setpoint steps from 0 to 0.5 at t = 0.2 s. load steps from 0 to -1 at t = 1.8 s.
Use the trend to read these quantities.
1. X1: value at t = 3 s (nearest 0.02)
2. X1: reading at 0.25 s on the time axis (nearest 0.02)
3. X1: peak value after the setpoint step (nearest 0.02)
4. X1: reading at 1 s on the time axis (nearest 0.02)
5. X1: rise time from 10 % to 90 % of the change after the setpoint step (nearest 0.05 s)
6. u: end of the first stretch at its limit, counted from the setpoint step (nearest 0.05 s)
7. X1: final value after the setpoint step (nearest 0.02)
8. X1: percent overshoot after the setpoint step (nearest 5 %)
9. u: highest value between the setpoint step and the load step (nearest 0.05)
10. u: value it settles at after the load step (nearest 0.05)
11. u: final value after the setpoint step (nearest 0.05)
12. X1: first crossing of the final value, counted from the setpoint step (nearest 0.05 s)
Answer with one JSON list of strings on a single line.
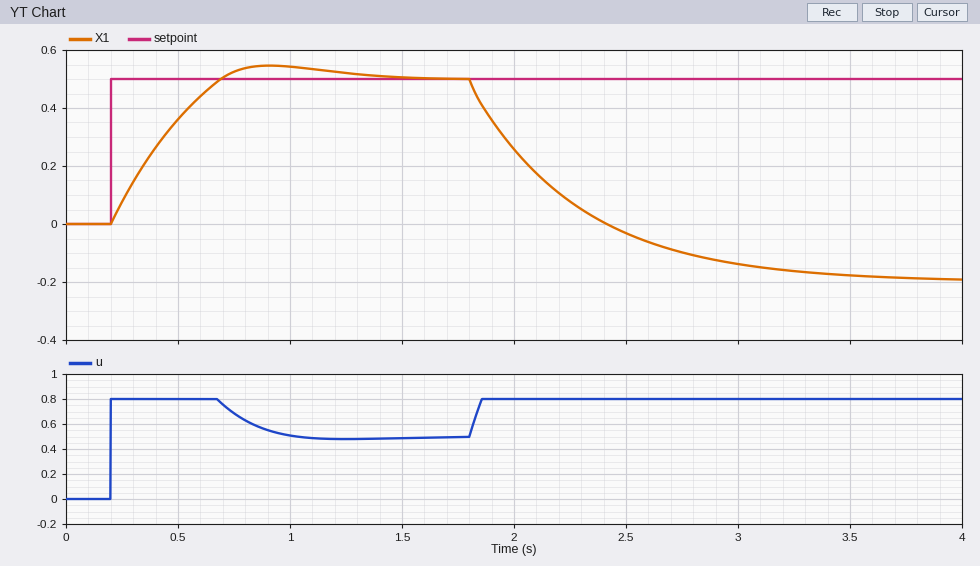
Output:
["-0.14", "0.08", "0.54", "0.54", "0.40 s", "0.50 s", "0.50", "10 %", "0.80", "0.80", "0.50", "0.50 s"]
